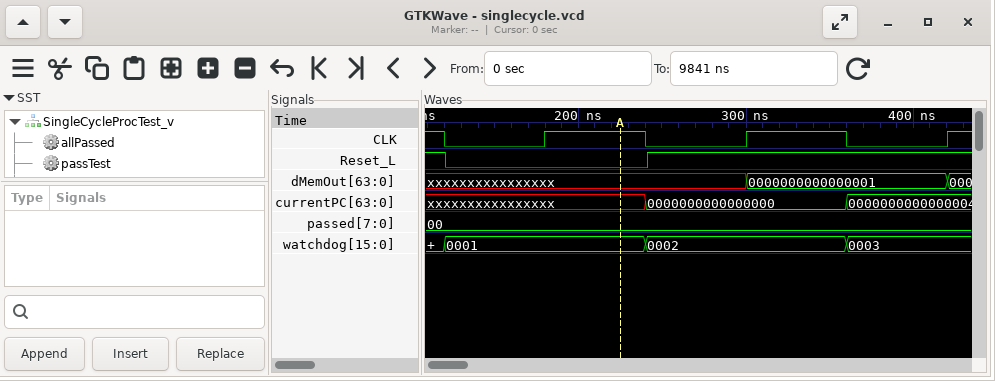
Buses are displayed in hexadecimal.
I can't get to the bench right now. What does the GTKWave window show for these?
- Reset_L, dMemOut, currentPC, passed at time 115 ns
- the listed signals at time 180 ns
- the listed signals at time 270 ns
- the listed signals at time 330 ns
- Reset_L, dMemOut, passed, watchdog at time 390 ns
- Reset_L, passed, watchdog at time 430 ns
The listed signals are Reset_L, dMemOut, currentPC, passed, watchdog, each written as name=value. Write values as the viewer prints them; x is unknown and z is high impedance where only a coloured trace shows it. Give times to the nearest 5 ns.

Reset_L=1, dMemOut=xxxxxxxxxxxxxxxx, currentPC=xxxxxxxxxxxxxxxx, passed=00
Reset_L=0, dMemOut=xxxxxxxxxxxxxxxx, currentPC=xxxxxxxxxxxxxxxx, passed=00, watchdog=0001
Reset_L=1, dMemOut=xxxxxxxxxxxxxxxx, currentPC=0000000000000000, passed=00, watchdog=0002
Reset_L=1, dMemOut=0000000000000001, currentPC=0000000000000000, passed=00, watchdog=0002
Reset_L=1, dMemOut=0000000000000001, passed=00, watchdog=0003
Reset_L=1, passed=00, watchdog=0003
